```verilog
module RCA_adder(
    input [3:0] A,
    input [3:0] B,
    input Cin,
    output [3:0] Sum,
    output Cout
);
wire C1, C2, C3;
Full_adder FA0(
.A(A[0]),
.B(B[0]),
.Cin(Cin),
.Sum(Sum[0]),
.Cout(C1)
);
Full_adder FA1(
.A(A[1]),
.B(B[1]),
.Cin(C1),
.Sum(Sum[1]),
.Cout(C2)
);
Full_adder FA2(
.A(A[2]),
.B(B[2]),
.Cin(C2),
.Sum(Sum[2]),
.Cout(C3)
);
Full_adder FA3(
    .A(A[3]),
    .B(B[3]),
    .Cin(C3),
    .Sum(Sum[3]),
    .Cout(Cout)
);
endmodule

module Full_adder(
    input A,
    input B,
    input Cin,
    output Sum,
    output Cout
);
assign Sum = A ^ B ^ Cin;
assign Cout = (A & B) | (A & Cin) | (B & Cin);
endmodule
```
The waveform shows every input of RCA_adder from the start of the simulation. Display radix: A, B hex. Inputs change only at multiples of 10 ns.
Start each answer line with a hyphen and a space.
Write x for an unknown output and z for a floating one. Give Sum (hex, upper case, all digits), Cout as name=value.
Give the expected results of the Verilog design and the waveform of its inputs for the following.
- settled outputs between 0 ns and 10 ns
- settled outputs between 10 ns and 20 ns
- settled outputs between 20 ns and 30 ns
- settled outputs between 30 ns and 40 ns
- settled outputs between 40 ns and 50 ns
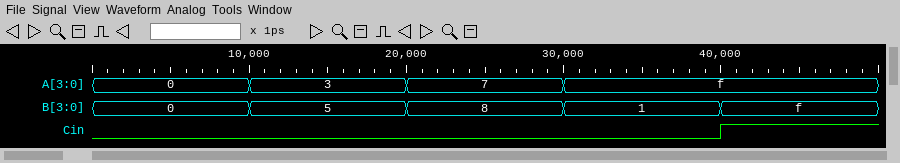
- Sum=0, Cout=0
- Sum=8, Cout=0
- Sum=F, Cout=0
- Sum=0, Cout=1
- Sum=F, Cout=1
